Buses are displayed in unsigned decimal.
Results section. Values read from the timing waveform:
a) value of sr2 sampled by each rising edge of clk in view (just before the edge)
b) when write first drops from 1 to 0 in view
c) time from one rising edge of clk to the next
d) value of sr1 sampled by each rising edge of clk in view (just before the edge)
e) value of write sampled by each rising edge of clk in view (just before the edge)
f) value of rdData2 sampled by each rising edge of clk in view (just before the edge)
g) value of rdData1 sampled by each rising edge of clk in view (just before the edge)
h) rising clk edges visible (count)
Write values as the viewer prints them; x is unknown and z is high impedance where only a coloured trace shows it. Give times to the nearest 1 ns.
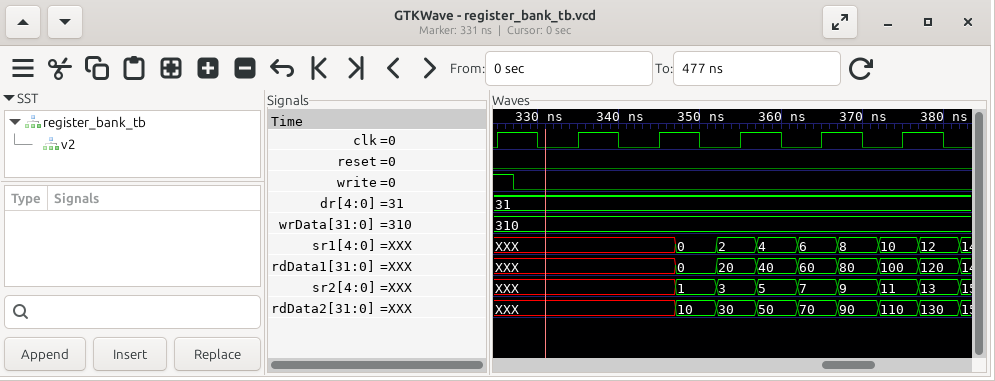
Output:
XXX, XXX, XXX, 3, 7, 11
327 ns
10 ns
XXX, XXX, XXX, 2, 6, 10
1 0 0 0 0 0
XXX, XXX, XXX, 30, 70, 110
XXX, XXX, XXX, 20, 60, 100
6
